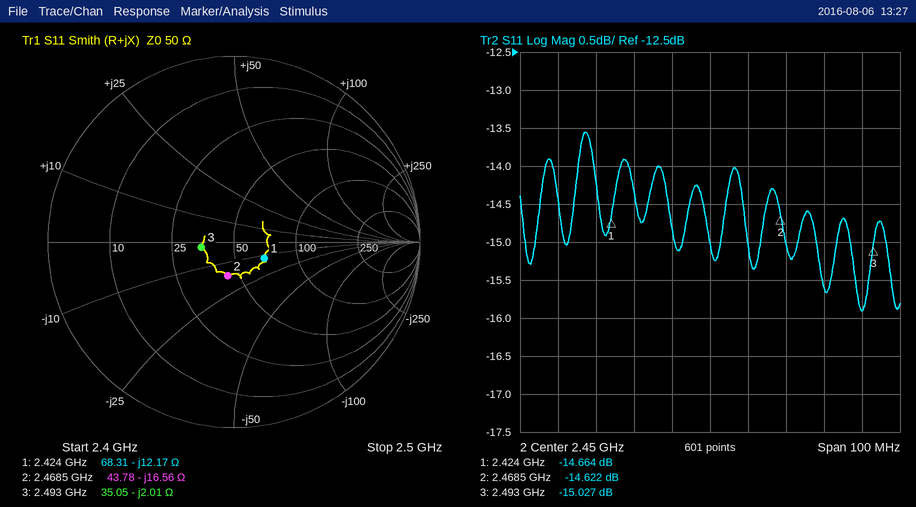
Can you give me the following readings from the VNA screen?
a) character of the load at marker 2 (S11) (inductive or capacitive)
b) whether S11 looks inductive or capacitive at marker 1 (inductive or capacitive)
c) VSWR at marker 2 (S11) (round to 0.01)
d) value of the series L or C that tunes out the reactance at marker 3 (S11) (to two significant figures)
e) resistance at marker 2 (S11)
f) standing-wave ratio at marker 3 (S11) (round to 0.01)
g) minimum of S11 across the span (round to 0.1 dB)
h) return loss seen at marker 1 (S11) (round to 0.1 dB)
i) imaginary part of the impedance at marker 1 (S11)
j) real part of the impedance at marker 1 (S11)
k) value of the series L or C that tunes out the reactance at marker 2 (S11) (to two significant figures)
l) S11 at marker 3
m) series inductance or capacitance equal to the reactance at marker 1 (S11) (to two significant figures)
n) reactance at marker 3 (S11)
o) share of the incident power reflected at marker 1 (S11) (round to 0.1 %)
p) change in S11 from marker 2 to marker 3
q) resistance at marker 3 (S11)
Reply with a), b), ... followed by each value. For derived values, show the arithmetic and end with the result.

a) capacitive
b) capacitive
c) 1.46
d) L = 2.01 Ω/(2π × 2.493 GHz) ≈ 128 pH, so 130 pH to two significant figures
e) 43.78 Ω
f) 1.43
g) -15.9 dB
h) 14.7 dB
i) -12.17 Ω
j) 68.31 Ω
k) L = 16.56 Ω/(2π × 2.4685 GHz) ≈ 1.1 nH
l) -15.027 dB
m) C = 1/(2π × 2.424 GHz × 12.17 Ω) ≈ 5.4 pF
n) -2.01 Ω
o) 10^(-14.664/10) ≈ 3.4 %
p) -15.027 − (-14.622) = -0.405 dB
q) 35.05 Ω
